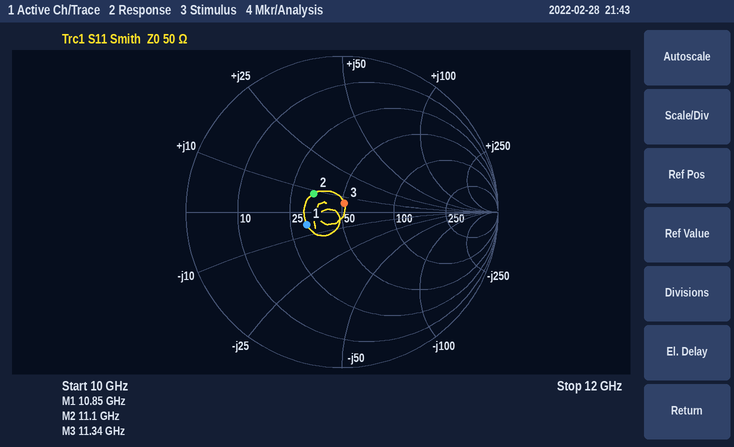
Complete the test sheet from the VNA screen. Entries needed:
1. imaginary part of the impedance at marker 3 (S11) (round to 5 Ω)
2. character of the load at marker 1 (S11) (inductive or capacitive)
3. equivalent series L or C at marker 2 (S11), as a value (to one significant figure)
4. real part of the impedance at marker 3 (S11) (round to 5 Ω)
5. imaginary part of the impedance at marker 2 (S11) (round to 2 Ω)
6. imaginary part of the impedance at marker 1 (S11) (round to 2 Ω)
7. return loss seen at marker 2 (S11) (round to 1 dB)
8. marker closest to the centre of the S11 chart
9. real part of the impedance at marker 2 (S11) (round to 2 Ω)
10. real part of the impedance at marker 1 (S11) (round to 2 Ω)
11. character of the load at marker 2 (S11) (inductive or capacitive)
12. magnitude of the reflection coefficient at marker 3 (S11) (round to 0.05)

+5 Ω
capacitive
100 pH
50 Ω
+8 Ω
-6 Ω
13 dB
marker 3
34 Ω
32 Ω
inductive
0.05
